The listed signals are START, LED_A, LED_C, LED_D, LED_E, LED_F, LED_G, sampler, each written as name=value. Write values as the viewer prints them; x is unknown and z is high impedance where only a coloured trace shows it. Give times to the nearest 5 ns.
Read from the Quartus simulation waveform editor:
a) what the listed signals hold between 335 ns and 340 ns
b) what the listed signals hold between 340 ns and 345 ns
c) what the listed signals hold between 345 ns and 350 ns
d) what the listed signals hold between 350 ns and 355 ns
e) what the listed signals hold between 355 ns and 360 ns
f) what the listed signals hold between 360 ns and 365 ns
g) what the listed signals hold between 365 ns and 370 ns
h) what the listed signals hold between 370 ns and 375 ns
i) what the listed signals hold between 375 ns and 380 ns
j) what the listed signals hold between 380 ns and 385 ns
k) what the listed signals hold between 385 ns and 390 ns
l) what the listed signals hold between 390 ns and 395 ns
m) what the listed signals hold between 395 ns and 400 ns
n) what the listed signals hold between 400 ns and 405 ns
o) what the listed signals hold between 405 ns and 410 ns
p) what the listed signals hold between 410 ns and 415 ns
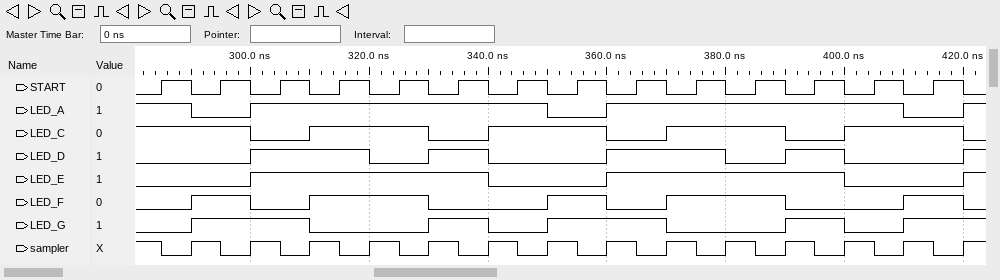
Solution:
START=1, LED_A=1, LED_C=0, LED_D=1, LED_E=1, LED_F=0, LED_G=1, sampler=0
START=0, LED_A=1, LED_C=1, LED_D=0, LED_E=0, LED_F=0, LED_G=0, sampler=1
START=1, LED_A=1, LED_C=1, LED_D=0, LED_E=0, LED_F=0, LED_G=0, sampler=0
START=0, LED_A=0, LED_C=1, LED_D=0, LED_E=0, LED_F=1, LED_G=1, sampler=1
START=1, LED_A=0, LED_C=1, LED_D=0, LED_E=0, LED_F=1, LED_G=1, sampler=0
START=0, LED_A=1, LED_C=0, LED_D=1, LED_E=1, LED_F=0, LED_G=1, sampler=1
START=1, LED_A=1, LED_C=0, LED_D=1, LED_E=1, LED_F=0, LED_G=1, sampler=0
START=0, LED_A=1, LED_C=1, LED_D=1, LED_E=1, LED_F=1, LED_G=0, sampler=1
START=1, LED_A=1, LED_C=1, LED_D=1, LED_E=1, LED_F=1, LED_G=0, sampler=0
START=0, LED_A=1, LED_C=1, LED_D=0, LED_E=1, LED_F=1, LED_G=0, sampler=1
START=1, LED_A=1, LED_C=1, LED_D=0, LED_E=1, LED_F=1, LED_G=0, sampler=0
START=0, LED_A=1, LED_C=0, LED_D=1, LED_E=1, LED_F=0, LED_G=1, sampler=1
START=1, LED_A=1, LED_C=0, LED_D=1, LED_E=1, LED_F=0, LED_G=1, sampler=0
START=0, LED_A=1, LED_C=1, LED_D=0, LED_E=0, LED_F=0, LED_G=0, sampler=1
START=1, LED_A=1, LED_C=1, LED_D=0, LED_E=0, LED_F=0, LED_G=0, sampler=0
START=0, LED_A=0, LED_C=1, LED_D=0, LED_E=0, LED_F=1, LED_G=1, sampler=1
